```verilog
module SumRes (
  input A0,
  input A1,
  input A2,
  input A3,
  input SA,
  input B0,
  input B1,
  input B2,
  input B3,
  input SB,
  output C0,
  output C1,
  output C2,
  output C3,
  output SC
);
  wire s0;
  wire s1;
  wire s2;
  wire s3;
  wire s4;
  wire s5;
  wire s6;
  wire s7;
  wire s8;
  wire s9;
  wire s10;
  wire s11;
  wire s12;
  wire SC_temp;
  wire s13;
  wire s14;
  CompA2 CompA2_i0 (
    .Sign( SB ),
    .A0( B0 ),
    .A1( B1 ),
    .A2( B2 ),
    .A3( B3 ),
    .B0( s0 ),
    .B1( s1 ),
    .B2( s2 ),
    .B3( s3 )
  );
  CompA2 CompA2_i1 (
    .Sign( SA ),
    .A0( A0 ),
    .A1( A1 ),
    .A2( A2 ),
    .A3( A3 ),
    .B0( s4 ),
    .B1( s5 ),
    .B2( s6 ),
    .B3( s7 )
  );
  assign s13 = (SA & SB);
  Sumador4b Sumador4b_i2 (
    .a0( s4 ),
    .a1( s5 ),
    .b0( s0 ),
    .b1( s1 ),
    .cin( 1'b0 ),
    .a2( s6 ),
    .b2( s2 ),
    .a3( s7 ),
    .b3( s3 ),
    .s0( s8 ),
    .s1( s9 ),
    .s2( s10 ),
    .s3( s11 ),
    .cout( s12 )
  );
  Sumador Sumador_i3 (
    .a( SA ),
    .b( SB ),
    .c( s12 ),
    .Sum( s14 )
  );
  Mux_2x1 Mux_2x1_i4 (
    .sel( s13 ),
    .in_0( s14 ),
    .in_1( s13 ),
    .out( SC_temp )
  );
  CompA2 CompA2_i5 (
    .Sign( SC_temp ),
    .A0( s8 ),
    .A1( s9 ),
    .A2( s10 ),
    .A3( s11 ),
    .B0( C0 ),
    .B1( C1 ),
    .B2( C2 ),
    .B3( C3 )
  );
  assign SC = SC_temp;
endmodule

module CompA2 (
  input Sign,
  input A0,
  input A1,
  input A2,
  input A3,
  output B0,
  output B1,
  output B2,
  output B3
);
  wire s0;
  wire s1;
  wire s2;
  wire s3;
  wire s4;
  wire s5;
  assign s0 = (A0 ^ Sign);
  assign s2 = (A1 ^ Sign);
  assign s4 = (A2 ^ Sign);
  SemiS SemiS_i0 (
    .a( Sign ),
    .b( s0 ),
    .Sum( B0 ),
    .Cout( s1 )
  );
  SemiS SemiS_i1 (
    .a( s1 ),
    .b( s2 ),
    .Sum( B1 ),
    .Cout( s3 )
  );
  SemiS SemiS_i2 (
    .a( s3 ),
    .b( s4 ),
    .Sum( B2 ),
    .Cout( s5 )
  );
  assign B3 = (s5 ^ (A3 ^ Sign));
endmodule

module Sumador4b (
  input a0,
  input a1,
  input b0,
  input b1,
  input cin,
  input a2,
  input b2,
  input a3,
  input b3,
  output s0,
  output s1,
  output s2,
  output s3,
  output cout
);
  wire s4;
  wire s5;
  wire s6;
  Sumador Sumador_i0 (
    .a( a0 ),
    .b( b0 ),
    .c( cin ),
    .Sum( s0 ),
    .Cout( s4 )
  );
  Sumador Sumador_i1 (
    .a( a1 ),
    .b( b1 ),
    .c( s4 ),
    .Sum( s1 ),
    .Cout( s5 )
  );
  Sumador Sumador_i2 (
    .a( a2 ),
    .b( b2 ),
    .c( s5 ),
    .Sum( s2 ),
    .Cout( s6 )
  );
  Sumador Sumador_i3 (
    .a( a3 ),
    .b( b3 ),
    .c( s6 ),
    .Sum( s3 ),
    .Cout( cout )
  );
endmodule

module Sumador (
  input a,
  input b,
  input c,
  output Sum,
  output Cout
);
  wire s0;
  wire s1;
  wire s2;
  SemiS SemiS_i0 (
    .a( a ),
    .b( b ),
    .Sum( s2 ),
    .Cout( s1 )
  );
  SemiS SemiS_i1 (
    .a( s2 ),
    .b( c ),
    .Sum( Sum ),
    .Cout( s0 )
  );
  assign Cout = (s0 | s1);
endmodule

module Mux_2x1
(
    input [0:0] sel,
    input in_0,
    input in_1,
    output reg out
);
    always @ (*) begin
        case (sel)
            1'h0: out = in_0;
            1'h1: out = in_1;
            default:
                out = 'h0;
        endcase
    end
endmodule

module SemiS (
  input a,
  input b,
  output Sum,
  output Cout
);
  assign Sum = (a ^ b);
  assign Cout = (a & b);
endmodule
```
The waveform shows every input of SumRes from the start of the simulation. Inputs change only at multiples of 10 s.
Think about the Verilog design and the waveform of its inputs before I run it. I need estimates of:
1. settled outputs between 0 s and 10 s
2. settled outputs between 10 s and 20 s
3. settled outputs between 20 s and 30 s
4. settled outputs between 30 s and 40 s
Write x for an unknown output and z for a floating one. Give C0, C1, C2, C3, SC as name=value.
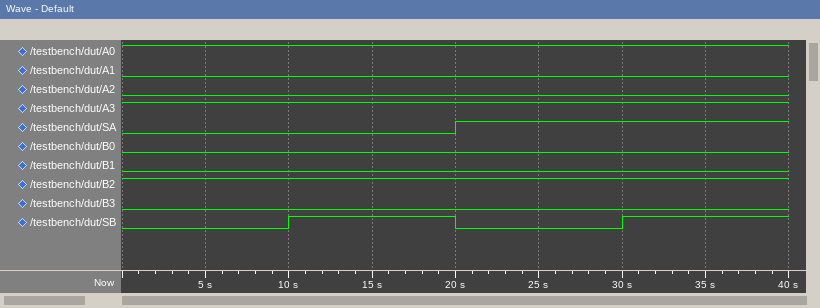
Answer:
C0=1, C1=0, C2=1, C3=1, SC=0
C0=1, C1=0, C2=1, C3=0, SC=0
C0=1, C1=0, C2=1, C3=0, SC=1
C0=1, C1=0, C2=1, C3=1, SC=1
